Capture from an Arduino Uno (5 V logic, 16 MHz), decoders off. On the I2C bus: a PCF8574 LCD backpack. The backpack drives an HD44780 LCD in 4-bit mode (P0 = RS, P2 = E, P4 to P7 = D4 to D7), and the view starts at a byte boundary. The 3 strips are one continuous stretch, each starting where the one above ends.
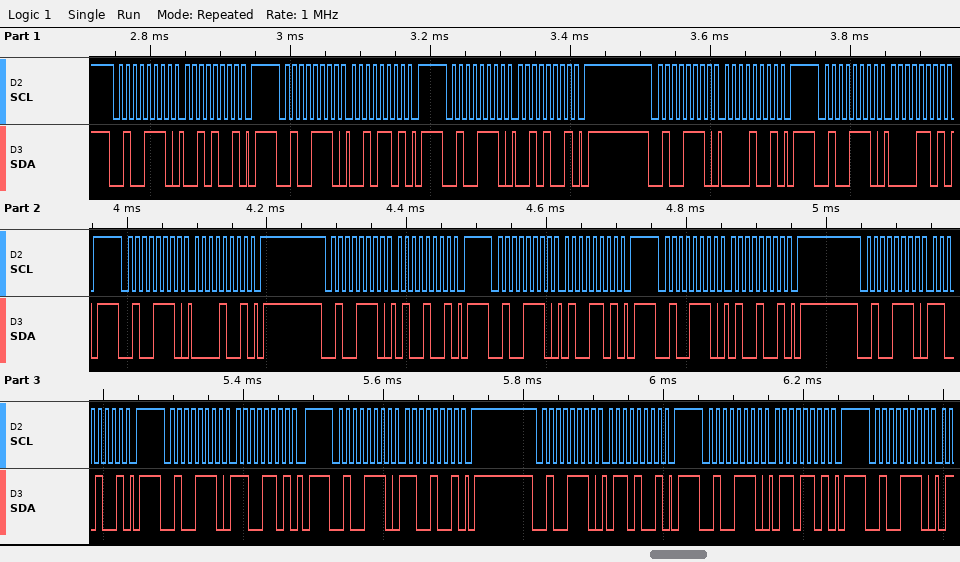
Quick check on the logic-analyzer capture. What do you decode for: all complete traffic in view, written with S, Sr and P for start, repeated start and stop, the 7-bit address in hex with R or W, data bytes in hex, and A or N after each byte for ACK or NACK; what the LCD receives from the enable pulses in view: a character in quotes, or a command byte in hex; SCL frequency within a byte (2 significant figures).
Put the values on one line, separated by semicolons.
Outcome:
S 27W A 29 A P S 27W A 2D A P S 27W A 29 A P S 27W A 09 A P S 27W A 0D A P S 27W A 09 A P S 27W A 49 A P S 27W A 4D A P S 27W A 49 A P S 27W A C9 A P S 27W A CD A P S 27W A C9 A P S 27W A 69 A P S 27W A 6D A P S 27W A; ' ' 'L'; 100 kHz
